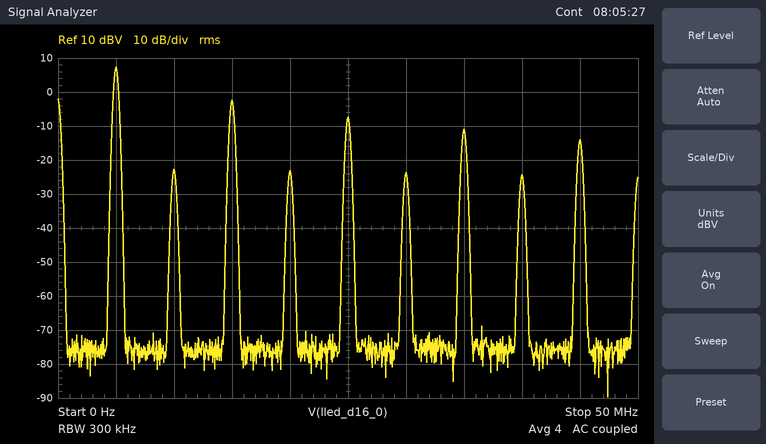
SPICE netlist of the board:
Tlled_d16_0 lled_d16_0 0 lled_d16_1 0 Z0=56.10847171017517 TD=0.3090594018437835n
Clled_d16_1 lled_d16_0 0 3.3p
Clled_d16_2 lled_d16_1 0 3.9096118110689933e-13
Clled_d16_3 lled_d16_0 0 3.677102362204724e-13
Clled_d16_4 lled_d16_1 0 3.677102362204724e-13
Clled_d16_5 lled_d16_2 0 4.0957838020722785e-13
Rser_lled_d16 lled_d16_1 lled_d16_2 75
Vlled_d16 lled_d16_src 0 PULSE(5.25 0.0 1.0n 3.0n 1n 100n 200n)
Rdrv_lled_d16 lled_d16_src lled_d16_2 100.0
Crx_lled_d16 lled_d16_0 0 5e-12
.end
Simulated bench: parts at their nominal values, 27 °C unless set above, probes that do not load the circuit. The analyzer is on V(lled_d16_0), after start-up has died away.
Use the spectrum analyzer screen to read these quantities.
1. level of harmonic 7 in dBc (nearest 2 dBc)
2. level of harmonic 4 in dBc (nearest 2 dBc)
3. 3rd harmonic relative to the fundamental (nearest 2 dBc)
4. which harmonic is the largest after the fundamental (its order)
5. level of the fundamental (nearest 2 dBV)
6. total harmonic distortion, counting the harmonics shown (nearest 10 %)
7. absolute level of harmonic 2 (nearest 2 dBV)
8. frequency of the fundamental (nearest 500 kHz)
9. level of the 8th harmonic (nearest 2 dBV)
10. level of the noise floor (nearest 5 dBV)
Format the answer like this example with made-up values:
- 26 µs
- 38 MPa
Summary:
- -18 dBc
- -30 dBc
- -10 dBc
- 3
- 8 dBV
- 40 %
- -22 dBV
- 5.0 MHz
- -24 dBV
- -75 dBV
